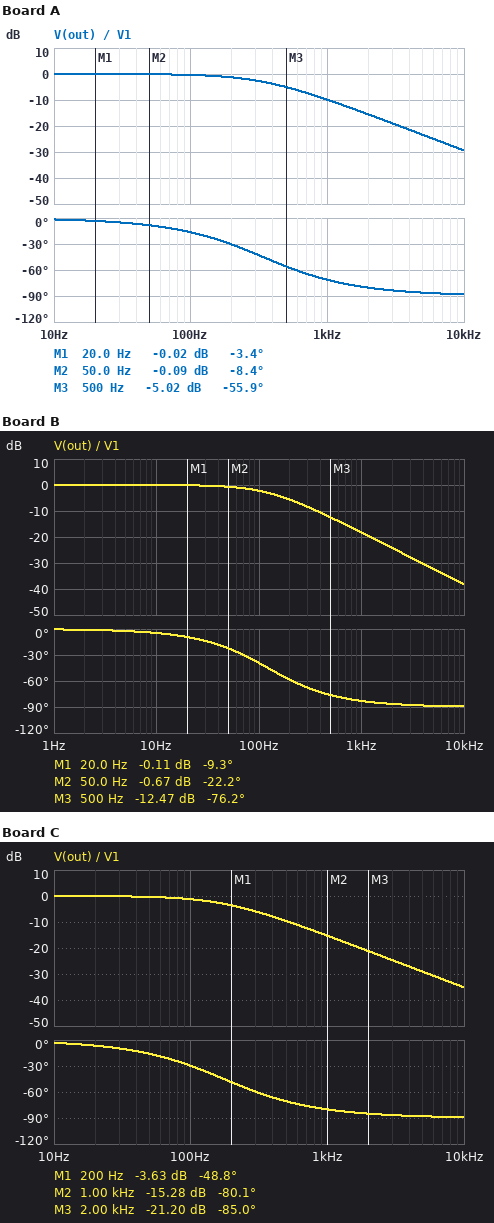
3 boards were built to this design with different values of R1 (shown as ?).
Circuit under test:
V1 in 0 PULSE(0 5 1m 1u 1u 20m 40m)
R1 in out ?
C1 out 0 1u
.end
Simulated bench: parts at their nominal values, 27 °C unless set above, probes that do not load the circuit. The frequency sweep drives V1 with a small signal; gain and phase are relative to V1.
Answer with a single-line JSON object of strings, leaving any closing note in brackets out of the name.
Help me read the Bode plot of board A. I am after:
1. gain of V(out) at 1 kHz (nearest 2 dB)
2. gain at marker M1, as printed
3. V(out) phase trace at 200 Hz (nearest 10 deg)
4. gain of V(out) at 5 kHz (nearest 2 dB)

{"gain of V(out) at 1 kHz": "-10 dB", "gain at marker M1, as printed": "-0.02 dB", "V(out) phase trace at 200 Hz": "-30 deg", "gain of V(out) at 5 kHz": "-24 dB"}
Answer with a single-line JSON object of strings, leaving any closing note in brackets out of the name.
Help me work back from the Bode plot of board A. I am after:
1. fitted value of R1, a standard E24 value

{"fitted value of R1, a standard E24 value": "470 Ω"}
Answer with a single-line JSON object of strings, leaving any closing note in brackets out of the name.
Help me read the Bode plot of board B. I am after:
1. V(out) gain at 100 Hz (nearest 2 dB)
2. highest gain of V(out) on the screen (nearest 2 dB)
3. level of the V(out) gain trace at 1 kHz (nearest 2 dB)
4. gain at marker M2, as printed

{"V(out) gain at 100 Hz": "-2 dB", "highest gain of V(out) on the screen": "0 dB", "level of the V(out) gain trace at 1 kHz": "-18 dB", "gain at marker M2, as printed": "-0.67 dB"}
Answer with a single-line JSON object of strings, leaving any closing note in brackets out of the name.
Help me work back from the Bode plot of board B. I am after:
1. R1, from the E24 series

{"R1, from the E24 series": "1.3 kΩ"}
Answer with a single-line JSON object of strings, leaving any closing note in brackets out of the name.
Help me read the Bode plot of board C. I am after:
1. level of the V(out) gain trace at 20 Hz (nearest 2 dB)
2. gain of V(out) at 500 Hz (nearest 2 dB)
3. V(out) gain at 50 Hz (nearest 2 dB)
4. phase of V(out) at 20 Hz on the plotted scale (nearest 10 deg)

{"level of the V(out) gain trace at 20 Hz": "0 dB", "gain of V(out) at 500 Hz": "-10 dB", "V(out) gain at 50 Hz": "0 dB", "phase of V(out) at 20 Hz on the plotted scale": "-10 deg"}
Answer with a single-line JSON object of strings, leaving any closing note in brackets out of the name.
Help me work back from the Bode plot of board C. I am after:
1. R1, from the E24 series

{"R1, from the E24 series": "910 Ω"}
